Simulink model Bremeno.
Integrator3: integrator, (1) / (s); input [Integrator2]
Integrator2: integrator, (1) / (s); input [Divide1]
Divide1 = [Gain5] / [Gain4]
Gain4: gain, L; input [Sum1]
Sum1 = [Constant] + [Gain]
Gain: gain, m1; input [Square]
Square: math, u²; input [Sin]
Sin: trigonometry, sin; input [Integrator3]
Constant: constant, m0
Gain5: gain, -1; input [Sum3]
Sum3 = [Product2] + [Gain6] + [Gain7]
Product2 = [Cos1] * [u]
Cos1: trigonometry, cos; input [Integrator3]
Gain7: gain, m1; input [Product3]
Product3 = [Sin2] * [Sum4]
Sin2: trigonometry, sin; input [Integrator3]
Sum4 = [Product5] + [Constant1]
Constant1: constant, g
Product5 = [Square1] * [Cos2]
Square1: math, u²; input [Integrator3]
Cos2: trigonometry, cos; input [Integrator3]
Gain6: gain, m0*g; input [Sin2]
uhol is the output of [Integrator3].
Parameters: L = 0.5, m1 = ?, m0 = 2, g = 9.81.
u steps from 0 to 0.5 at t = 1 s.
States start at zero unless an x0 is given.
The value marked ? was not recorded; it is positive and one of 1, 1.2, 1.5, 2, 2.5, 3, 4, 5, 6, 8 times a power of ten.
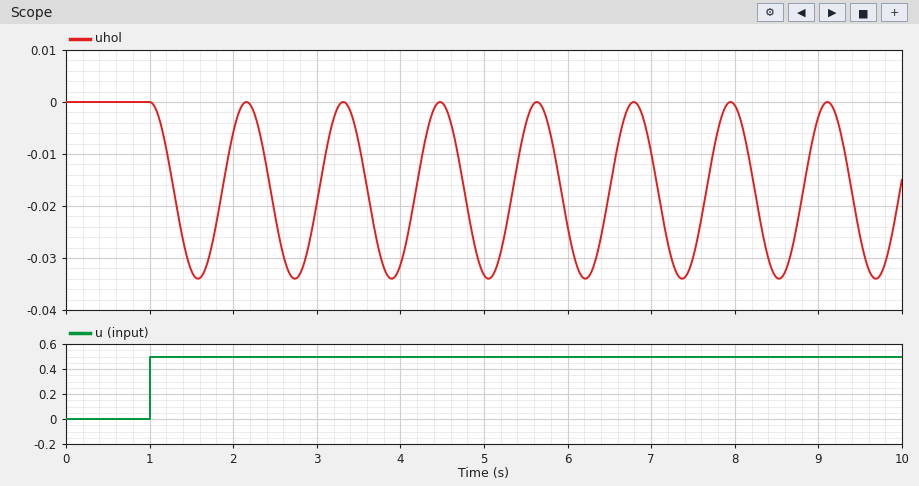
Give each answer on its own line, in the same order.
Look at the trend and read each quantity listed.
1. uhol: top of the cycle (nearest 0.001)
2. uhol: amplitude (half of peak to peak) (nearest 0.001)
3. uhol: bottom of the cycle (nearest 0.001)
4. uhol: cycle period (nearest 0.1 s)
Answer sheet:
0.000
0.017
-0.034
1.2 s
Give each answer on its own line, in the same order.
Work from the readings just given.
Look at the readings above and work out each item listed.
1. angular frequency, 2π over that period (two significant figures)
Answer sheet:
5.2 rad/s
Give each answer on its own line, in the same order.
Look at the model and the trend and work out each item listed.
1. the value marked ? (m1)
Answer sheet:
1
